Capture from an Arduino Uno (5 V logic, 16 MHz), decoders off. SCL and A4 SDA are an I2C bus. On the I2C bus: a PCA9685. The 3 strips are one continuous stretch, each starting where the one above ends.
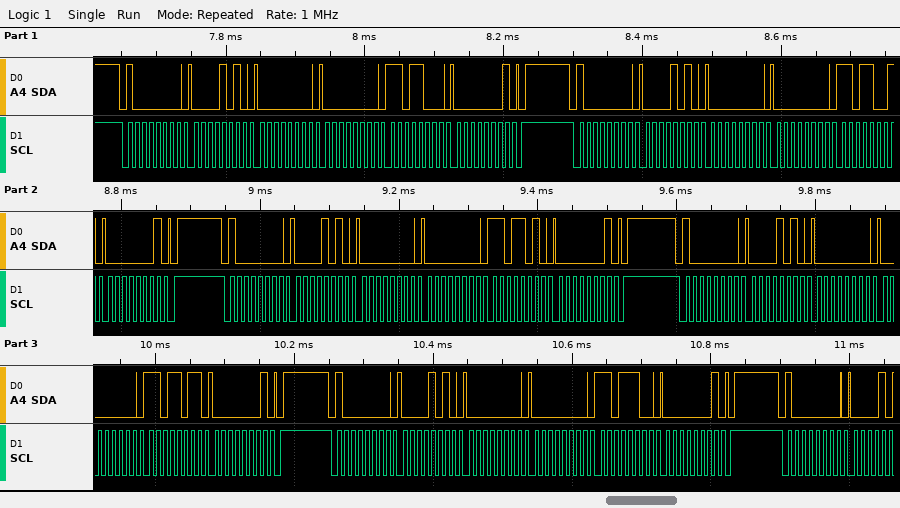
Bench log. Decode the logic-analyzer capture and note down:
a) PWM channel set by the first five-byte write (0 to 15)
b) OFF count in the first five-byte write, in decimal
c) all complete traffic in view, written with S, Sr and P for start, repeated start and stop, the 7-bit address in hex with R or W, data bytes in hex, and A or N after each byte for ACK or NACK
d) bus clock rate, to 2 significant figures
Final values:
1
472
S 40W A 0A A 00 A 00 A D8 A 01 A P S 40W A 0A A 00 A 00 A D9 A 01 A P S 40W A 0A A 00 A 00 A DA A 01 A P S 40W A 0A A 00 A 00 A DB A 01 A P S 40W A 0A A 00 A 00 A DC A 01 A P S 40W A
100 kHz
